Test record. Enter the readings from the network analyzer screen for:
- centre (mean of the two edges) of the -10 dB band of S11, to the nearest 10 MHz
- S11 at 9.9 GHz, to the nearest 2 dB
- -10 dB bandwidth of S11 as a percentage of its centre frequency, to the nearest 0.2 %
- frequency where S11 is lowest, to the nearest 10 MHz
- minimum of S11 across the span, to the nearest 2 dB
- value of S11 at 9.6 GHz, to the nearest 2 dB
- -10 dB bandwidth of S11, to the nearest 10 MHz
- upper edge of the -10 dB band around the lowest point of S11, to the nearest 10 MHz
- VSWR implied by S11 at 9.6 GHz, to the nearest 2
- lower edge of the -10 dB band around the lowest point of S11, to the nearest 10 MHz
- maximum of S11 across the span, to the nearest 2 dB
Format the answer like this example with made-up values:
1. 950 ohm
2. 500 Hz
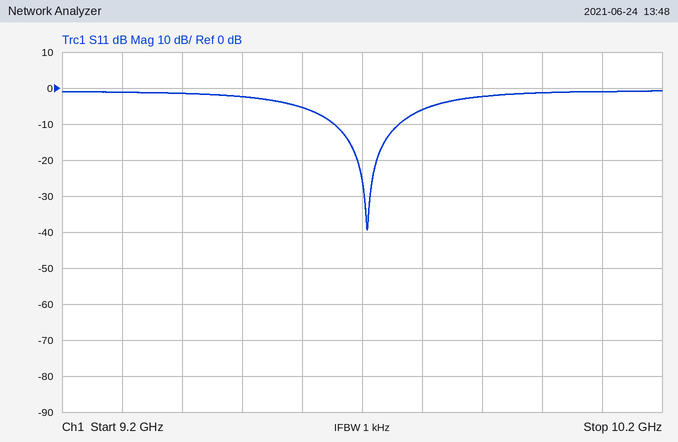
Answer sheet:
1. 9.71 GHz
2. -2 dB
3. 1.2 %
4. 9.71 GHz
5. -40 dB
6. -6 dB
7. 110 MHz
8. 9.76 GHz
9. 4
10. 9.65 GHz
11. 0 dB
